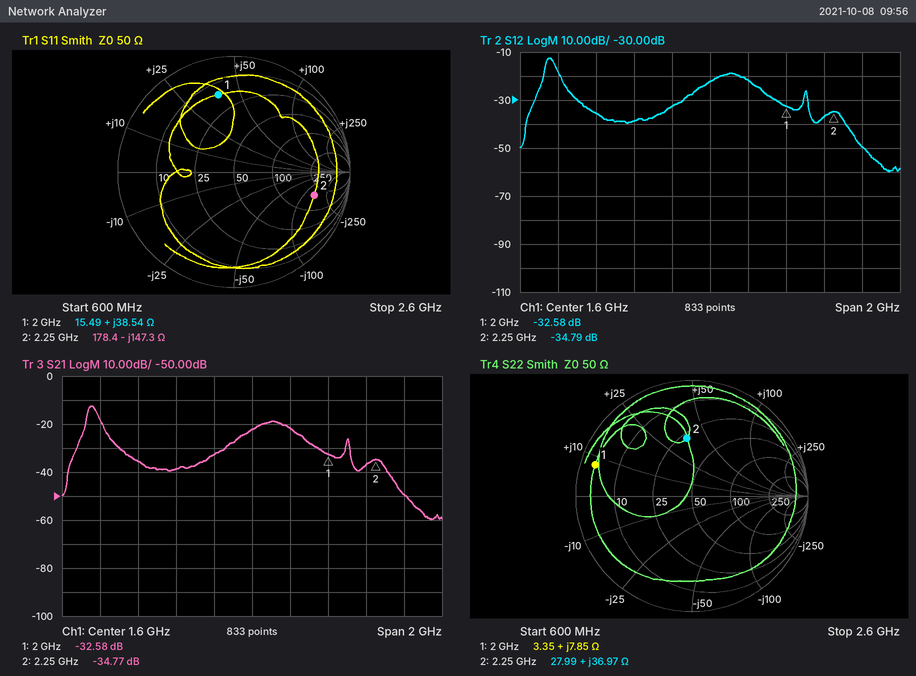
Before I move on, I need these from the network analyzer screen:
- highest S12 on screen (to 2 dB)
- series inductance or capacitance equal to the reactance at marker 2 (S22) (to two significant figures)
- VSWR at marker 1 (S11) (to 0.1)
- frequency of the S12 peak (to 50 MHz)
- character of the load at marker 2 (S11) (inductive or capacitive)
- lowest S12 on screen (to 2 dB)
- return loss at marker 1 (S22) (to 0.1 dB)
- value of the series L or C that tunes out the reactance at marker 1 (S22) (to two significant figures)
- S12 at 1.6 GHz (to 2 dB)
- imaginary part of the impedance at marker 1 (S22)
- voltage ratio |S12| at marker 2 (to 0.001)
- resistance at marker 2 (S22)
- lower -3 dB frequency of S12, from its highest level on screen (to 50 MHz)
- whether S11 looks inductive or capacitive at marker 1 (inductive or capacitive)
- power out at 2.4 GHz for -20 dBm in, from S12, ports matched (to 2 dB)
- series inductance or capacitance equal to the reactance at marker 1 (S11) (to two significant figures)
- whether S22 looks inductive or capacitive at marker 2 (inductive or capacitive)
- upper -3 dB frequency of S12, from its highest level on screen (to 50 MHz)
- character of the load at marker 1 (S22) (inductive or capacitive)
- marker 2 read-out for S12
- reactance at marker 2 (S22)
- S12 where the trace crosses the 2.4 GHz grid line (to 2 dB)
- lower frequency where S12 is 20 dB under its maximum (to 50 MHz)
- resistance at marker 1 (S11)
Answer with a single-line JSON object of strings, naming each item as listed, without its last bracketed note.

{"highest S12 on screen": "-12 dB", "series inductance or capacitance equal to the reactance at marker 2 (S22)": "2.6 nH", "VSWR at marker 1 (S11)": "5.3", "frequency of the S12 peak": "750 MHz", "character of the load at marker 2 (S11)": "capacitive", "lowest S12 on screen": "-60 dB", "return loss at marker 1 (S22)": "1.1 dB", "value of the series L or C that tunes out the reactance at marker 1 (S22)": "10 pF", "S12 at 1.6 GHz": "-22 dB", "imaginary part of the impedance at marker 1": "+7.85 Ω", "voltage ratio |S12| at marker 2": "0.018", "resistance at marker 2": "27.99 Ω", "lower -3 dB frequency of S12, from its highest level on screen": "750 MHz", "whether S11 looks inductive or capacitive at marker 1": "inductive", "power out at 2.4 GHz for -20 dBm in, from S12, ports matched": "-70 dBm", "series inductance or capacitance equal to the reactance at marker 1 (S11)": "3.1 nH", "whether S22 looks inductive or capacitive at marker 2": "inductive", "upper -3 dB frequency of S12, from its highest level on screen": "800 MHz", "character of the load at marker 1 (S22)": "inductive", "marker 2 read-out for S12": "-34.79 dB", "reactance at marker 2": "+36.97 Ω", "S12 where the trace crosses the 2.4 GHz grid line": "-50 dB", "lower frequency where S12 is 20 dB under its maximum": "650 MHz", "resistance at marker 1": "15.49 Ω"}
